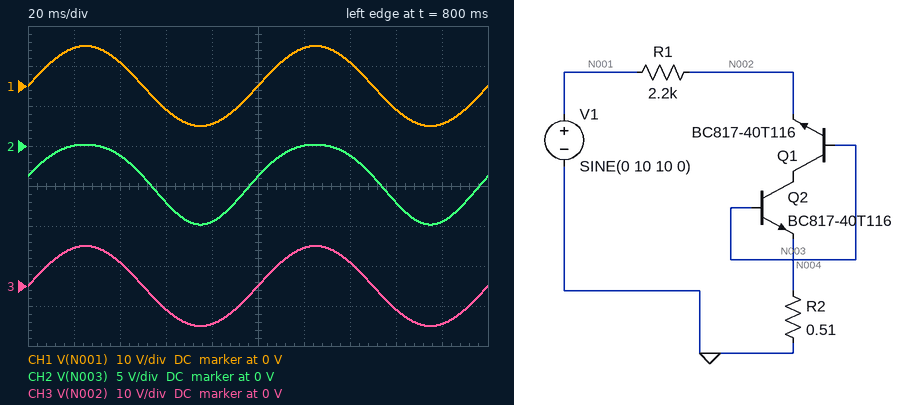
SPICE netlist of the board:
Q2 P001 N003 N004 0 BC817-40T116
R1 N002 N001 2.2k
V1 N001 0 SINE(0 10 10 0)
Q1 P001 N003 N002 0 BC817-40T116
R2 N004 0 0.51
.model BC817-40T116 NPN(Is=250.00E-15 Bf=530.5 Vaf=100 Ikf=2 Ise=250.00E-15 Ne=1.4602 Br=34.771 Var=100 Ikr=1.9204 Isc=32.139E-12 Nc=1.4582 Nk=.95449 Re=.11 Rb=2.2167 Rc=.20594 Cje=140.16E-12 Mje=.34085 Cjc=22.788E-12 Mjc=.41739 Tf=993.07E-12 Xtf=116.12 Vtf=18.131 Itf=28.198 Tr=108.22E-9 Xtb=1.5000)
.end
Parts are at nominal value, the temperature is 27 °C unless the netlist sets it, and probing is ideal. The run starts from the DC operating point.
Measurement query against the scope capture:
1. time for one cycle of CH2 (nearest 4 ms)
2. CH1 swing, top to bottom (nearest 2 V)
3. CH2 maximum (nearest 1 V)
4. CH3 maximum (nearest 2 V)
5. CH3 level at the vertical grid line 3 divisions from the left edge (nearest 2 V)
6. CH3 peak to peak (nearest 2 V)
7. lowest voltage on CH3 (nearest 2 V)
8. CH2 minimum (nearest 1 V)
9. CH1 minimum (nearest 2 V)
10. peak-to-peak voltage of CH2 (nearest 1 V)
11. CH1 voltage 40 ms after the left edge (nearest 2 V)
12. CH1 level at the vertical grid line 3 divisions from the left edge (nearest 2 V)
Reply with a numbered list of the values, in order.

1. 100 ms
2. 20 V
3. 0 V
4. 10 V
5. -6 V
6. 20 V
7. -10 V
8. -10 V
9. -10 V
10. 10 V
11. 6 V
12. -6 V
